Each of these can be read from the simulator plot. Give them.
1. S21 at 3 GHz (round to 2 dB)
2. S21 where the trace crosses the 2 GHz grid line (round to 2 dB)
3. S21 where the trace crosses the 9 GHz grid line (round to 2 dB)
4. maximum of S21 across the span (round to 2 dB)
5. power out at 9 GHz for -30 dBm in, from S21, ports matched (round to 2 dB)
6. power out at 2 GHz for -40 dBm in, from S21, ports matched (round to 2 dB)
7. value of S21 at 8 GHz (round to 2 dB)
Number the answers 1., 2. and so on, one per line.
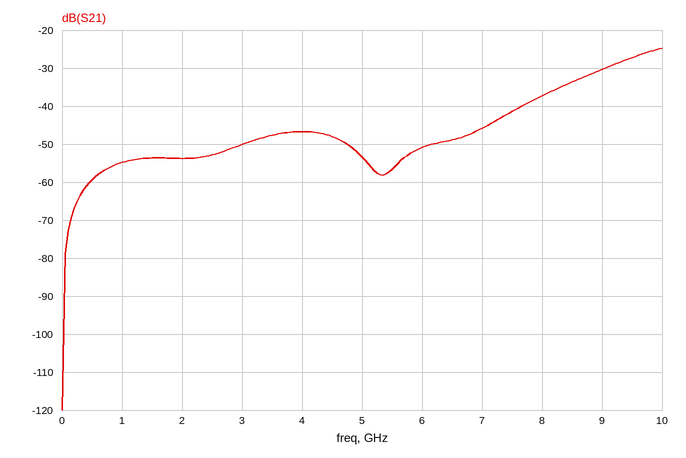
1. -50 dB
2. -54 dB
3. -30 dB
4. -24 dB
5. -60 dBm
6. -94 dBm
7. -38 dB
